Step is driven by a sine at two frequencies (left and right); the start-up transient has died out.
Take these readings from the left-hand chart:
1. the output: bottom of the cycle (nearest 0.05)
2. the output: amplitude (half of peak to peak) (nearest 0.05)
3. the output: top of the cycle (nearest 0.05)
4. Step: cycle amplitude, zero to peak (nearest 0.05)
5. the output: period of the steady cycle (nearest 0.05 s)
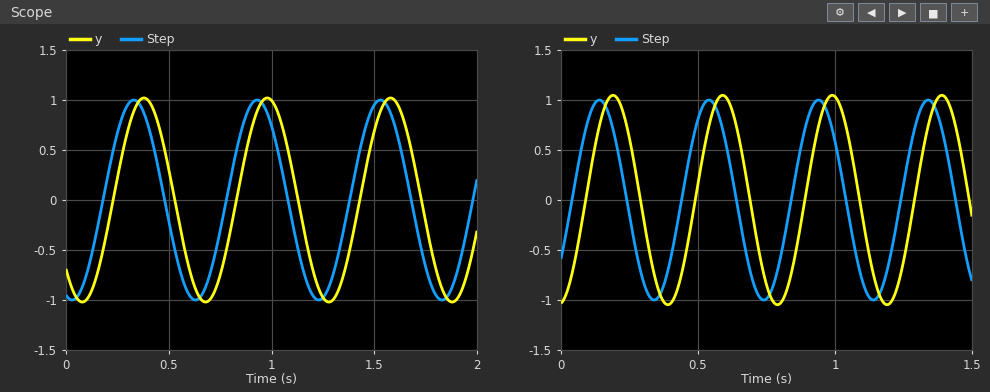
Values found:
-1.00
1.00
1.00
1.00
0.60 s
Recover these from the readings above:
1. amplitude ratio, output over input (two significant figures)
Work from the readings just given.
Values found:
1.0
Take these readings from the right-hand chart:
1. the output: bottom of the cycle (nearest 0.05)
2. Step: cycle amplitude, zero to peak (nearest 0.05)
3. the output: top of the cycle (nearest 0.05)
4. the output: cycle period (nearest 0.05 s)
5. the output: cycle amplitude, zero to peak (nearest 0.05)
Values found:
-1.05
1.00
1.05
0.40 s
1.05
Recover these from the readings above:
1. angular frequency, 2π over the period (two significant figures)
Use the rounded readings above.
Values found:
16 rad/s
